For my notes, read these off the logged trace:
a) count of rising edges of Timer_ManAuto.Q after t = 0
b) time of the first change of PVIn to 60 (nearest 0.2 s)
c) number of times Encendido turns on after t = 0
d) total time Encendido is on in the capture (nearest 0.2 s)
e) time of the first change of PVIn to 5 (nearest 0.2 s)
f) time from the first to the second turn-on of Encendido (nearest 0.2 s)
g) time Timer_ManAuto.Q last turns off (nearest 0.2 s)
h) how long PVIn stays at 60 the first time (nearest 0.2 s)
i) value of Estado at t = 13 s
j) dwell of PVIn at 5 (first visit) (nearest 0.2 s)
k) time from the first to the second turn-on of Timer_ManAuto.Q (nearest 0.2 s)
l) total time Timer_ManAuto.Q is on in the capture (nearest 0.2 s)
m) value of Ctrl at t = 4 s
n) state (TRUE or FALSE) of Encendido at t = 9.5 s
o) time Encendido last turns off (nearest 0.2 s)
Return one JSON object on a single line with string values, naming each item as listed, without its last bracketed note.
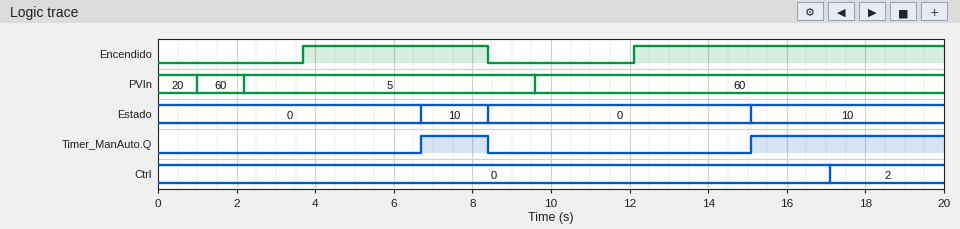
{"count of rising edges of Timer_ManAuto.Q after t = 0": "2", "time of the first change of PVIn to 60": "1.0 s", "number of times Encendido turns on after t = 0": "2", "total time Encendido is on in the capture": "12.6 s", "time of the first change of PVIn to 5": "2.2 s", "time from the first to the second turn-on of Encendido": "8.4 s", "time Timer_ManAuto.Q last turns off": "8.4 s", "how long PVIn stays at 60 the first time": "1.2 s", "value of Estado at t = 13 s": "0", "dwell of PVIn at 5 (first visit)": "7.4 s", "time from the first to the second turn-on of Timer_ManAuto.Q": "8.4 s", "total time Timer_ManAuto.Q is on in the capture": "6.6 s", "value of Ctrl at t = 4 s": "0", "state (TRUE or FALSE) of Encendido at t = 9.5 s": "FALSE", "time Encendido last turns off": "8.4 s"}
